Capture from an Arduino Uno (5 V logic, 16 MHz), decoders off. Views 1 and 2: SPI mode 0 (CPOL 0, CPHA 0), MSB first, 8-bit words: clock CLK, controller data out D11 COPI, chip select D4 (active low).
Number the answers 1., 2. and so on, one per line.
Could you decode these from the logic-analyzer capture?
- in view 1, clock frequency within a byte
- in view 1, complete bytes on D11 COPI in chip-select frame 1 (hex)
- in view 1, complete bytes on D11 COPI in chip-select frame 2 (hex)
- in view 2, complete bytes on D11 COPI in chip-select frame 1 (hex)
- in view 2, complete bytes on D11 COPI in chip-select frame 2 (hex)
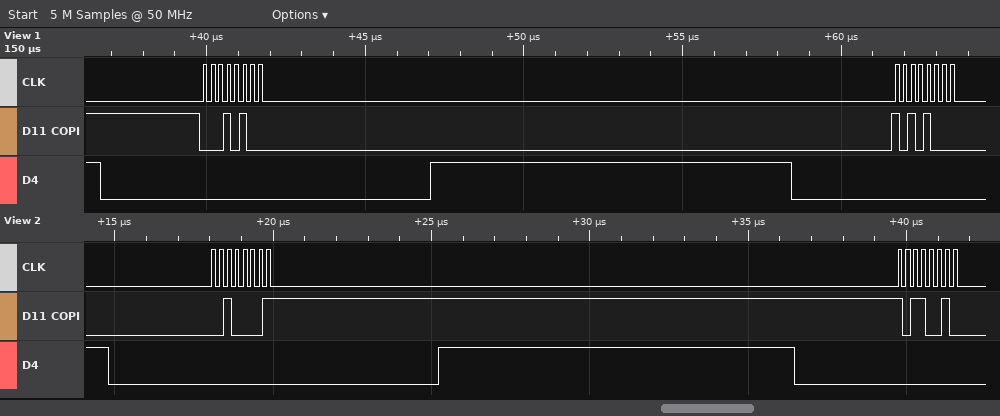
1. 4 MHz
2. 14
3. A8
4. 21
5. B2
